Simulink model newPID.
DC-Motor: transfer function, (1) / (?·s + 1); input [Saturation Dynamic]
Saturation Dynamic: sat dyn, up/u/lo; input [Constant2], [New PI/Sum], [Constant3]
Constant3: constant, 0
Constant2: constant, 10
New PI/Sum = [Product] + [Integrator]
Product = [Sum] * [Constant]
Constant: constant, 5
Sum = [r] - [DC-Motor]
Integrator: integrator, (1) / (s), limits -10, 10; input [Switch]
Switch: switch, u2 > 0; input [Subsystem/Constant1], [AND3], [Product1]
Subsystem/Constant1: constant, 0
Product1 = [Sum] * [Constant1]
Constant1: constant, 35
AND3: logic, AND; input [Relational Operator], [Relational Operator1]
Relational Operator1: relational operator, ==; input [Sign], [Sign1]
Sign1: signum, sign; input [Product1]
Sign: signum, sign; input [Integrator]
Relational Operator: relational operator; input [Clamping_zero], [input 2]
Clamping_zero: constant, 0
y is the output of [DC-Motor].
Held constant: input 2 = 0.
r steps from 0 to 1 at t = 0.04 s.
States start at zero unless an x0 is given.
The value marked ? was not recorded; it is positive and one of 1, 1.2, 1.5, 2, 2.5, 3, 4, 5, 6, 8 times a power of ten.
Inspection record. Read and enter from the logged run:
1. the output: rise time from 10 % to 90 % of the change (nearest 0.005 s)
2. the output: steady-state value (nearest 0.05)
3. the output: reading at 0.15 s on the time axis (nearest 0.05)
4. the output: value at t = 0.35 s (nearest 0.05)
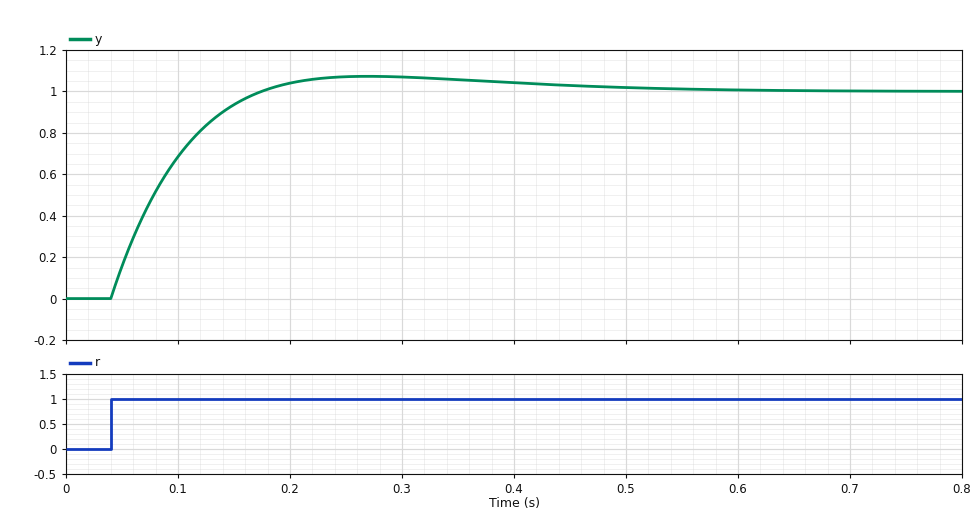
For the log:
0.095 s
1.00
0.95
1.05
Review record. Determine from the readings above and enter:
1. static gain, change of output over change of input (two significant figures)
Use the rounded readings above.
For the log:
1.0
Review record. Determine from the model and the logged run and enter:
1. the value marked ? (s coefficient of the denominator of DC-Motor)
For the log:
0.3
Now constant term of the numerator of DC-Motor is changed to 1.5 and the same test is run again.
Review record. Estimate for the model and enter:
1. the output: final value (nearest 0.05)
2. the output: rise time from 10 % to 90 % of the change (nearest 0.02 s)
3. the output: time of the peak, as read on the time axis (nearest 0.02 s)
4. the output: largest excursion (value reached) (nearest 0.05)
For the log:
1.00
0.06 s
0.22 s
1.05
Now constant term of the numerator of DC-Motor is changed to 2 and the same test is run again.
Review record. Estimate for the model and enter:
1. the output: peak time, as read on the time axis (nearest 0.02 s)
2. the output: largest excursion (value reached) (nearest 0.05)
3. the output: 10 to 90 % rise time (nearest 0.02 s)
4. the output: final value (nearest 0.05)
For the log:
0.18 s
1.05
0.06 s
1.00
